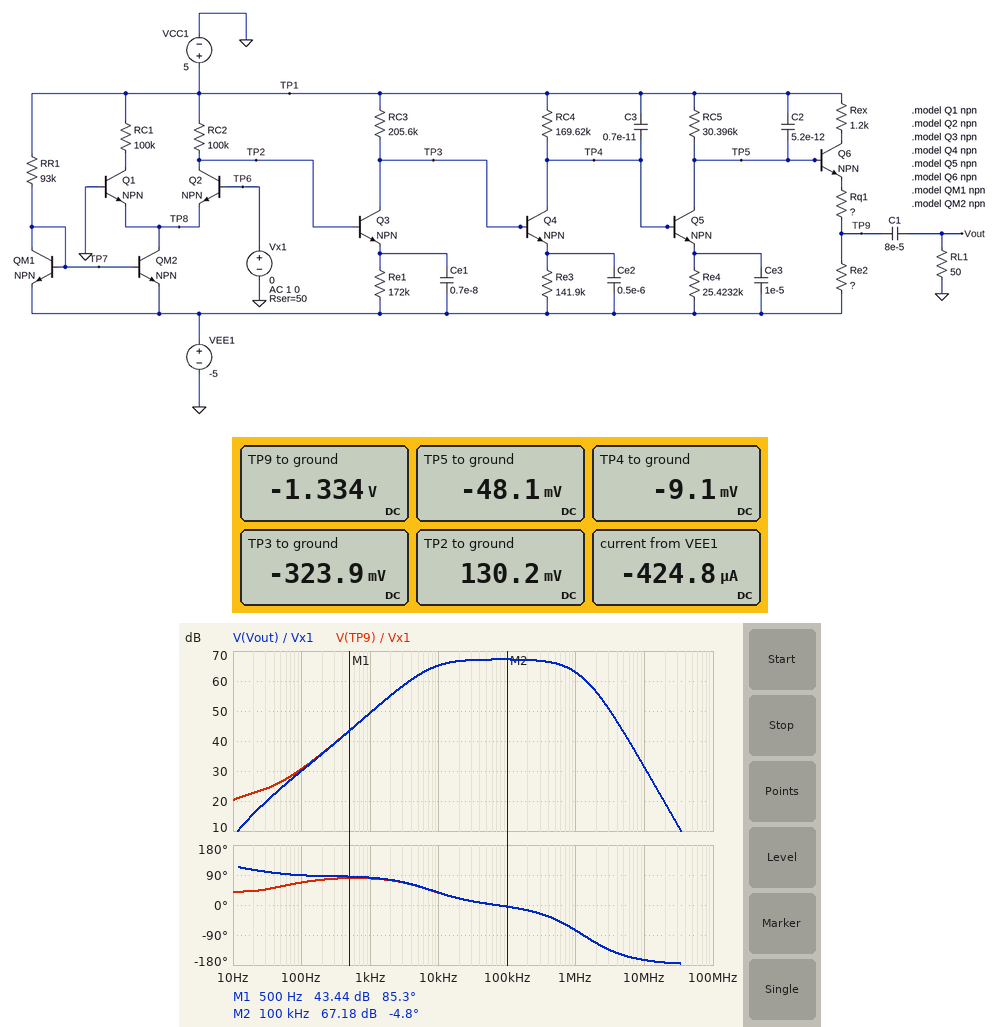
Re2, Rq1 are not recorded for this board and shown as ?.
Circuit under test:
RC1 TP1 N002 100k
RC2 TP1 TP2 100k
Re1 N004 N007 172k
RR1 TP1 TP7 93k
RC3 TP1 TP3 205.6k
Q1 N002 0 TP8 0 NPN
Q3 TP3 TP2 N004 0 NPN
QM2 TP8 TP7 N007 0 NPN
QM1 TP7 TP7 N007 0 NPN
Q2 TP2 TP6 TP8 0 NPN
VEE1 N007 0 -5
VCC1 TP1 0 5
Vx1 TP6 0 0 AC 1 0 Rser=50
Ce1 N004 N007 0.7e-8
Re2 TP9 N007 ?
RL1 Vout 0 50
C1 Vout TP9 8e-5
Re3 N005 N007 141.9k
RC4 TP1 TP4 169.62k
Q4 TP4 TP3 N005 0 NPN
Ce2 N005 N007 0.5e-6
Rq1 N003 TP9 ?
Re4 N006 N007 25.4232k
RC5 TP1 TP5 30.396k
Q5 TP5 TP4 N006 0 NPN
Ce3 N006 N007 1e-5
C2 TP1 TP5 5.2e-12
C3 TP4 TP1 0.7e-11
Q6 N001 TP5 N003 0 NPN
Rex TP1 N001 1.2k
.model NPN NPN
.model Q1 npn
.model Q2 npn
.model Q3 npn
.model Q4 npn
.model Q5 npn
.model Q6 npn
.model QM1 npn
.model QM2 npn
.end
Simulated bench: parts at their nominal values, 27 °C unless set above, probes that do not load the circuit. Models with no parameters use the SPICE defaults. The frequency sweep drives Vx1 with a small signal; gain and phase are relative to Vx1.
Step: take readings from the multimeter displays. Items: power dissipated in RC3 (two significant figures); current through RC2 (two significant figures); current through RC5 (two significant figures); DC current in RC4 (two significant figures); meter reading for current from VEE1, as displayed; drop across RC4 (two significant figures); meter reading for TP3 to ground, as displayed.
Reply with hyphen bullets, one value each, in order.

- 140 µW
- 49 µA
- 170 µA
- 30 µA
- -424.8 µA
- 5.0 V
- -323.9 mV
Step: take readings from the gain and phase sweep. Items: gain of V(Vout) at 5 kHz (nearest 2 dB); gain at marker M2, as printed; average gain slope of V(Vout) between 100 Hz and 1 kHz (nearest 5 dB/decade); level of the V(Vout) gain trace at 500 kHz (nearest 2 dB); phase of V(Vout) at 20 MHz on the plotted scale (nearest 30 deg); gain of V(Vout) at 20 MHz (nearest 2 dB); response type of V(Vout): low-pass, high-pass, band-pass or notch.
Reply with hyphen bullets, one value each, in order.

- 62 dB
- 67.18 dB
- 20 dB/decade
- 66 dB
- -180 deg
- 20 dB
- band-pass
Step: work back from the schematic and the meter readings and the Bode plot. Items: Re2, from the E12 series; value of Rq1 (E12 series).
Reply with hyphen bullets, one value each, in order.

- 680 kΩ
- 120 kΩ
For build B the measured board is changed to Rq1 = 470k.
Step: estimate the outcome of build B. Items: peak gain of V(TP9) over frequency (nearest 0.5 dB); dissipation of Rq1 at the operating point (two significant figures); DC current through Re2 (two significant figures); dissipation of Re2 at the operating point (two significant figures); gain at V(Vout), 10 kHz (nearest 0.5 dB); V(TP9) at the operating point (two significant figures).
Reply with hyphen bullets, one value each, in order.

- 55.5 dB
- 6.6 µW
- 3.8 µA
- 9.6 µW
- 53.5 dB
- -2.4 V
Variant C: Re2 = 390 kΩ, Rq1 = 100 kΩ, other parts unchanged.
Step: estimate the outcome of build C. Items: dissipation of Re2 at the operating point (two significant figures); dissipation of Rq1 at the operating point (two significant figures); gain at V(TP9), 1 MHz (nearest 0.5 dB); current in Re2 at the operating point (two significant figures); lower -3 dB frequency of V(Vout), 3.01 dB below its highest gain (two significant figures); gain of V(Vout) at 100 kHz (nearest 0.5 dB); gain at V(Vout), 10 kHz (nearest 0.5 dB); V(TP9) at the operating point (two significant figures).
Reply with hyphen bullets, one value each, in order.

- 30 µW
- 7.7 µW
- 64.5 dB
- 8.8 µA
- 7.7 kHz
- 69.0 dB
- 67.0 dB
- -1.6 V
